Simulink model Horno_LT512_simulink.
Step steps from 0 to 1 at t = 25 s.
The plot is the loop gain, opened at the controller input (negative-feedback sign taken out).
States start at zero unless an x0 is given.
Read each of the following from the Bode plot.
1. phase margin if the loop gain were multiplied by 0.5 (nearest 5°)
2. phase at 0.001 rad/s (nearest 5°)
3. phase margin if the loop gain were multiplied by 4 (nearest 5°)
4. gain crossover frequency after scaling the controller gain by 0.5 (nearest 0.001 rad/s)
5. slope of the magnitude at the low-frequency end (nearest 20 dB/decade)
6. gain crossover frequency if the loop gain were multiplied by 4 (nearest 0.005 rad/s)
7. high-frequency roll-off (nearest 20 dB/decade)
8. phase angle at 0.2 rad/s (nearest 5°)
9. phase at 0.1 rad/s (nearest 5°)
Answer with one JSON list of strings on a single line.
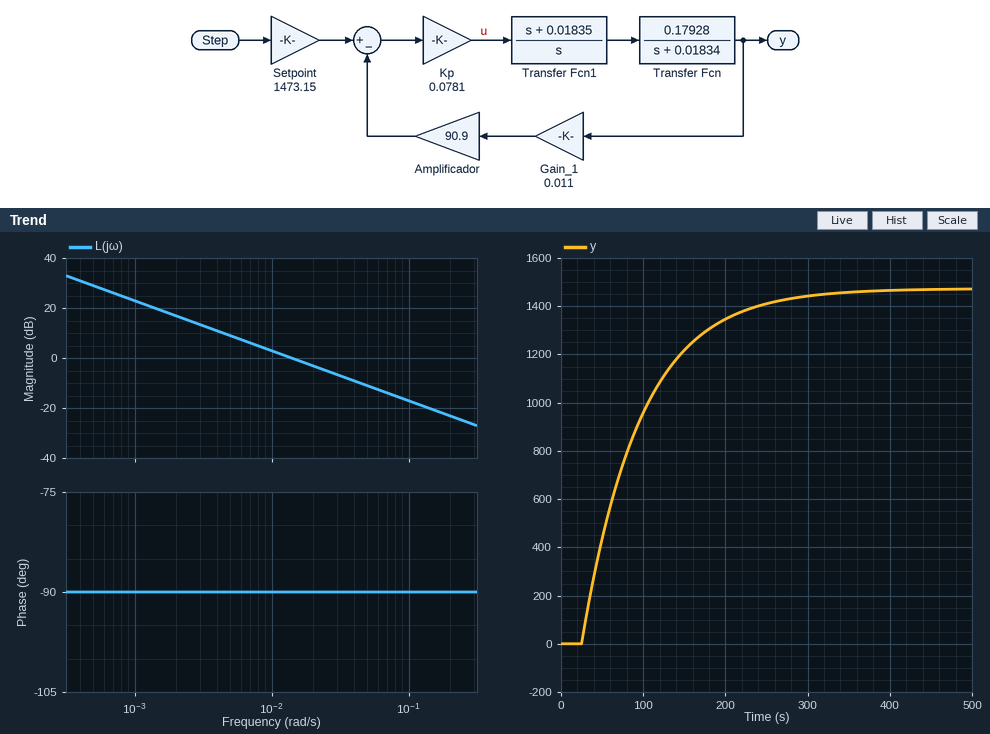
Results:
["90°", "-90°", "90°", "0.007 rad/s", "-20 dB/decade", "0.055 rad/s", "-20 dB/decade", "-90°", "-90°"]
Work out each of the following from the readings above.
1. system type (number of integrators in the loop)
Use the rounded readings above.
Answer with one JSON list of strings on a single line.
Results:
["1"]
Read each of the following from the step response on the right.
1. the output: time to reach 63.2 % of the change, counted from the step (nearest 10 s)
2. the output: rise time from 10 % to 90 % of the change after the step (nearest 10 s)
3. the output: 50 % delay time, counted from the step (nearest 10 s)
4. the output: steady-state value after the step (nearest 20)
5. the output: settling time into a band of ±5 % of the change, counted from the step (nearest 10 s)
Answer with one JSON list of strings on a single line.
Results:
["70 s", "160 s", "50 s", "1480", "210 s"]
